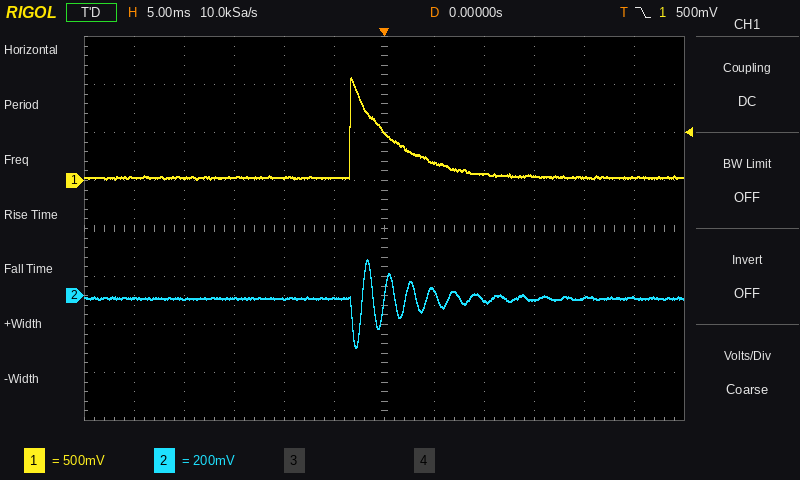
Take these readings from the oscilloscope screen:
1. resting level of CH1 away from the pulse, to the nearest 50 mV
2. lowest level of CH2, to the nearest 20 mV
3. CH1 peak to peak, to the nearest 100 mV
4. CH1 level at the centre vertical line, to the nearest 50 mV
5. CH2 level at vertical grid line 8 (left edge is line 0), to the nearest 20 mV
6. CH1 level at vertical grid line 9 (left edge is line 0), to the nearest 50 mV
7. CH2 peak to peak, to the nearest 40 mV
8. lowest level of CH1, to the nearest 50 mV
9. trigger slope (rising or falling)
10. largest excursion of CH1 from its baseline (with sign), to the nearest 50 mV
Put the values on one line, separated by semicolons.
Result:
50 mV; -220 mV; 1.10 V; 500 mV; -20 mV; 50 mV; 360 mV; 0 mV; falling; +1.05 V
